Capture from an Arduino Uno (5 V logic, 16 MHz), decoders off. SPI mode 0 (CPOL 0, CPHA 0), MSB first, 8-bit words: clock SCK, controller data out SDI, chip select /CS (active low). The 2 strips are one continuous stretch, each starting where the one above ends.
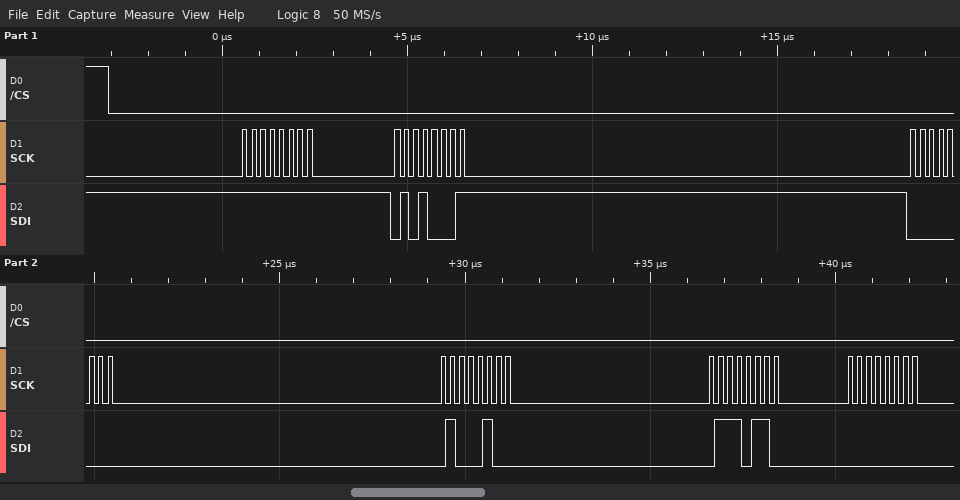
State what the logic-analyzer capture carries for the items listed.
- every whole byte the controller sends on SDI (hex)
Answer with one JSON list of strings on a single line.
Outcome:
["FF 51 00 44 76 00"]
